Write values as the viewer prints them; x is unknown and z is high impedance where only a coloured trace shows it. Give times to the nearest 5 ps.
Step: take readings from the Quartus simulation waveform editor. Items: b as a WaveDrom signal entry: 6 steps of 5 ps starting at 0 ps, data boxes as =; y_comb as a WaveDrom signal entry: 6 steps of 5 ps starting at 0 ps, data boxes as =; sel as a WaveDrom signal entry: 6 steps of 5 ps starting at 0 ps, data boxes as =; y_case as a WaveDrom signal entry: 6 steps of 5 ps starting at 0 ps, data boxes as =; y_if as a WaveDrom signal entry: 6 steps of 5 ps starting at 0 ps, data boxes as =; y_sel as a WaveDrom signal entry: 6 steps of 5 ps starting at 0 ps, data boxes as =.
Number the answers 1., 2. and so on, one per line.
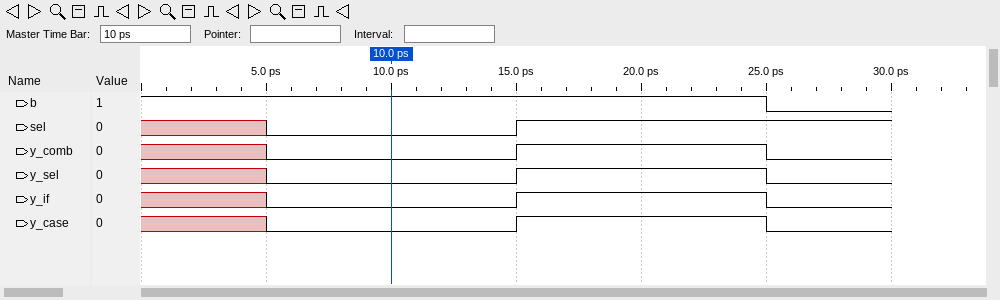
1. {name: 'b', wave: '1....0'}
2. {name: 'y_comb', wave: 'x0.1.0'}
3. {name: 'sel', wave: 'x0.1..'}
4. {name: 'y_case', wave: 'x0.1.0'}
5. {name: 'y_if', wave: 'x0.1.0'}
6. {name: 'y_sel', wave: 'x0.1.0'}
